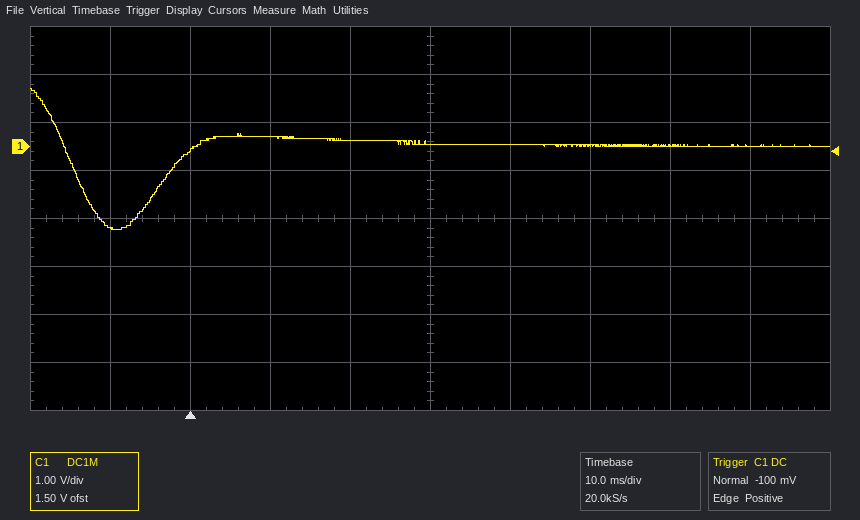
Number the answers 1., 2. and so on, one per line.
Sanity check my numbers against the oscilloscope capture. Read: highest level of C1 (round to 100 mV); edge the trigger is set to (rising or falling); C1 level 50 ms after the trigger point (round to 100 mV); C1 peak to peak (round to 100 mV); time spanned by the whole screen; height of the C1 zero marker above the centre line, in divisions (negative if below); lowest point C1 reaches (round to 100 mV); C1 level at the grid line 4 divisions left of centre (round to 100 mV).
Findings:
1. 1.2 V
2. rising
3. 0.0 V
4. 2.9 V
5. 100 ms
6. +1.5 div
7. -1.7 V
8. -1.7 V
